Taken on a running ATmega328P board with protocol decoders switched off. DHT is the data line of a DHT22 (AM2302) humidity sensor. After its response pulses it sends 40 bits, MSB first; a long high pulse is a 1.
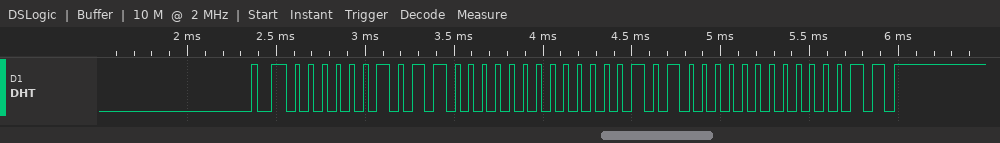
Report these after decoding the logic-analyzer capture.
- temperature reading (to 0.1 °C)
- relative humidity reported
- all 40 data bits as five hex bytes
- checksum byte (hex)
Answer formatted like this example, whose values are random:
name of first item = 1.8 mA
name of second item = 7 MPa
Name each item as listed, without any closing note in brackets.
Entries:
temperature reading = 32.0 °C
relative humidity reported = 70.4 %
all 40 data bits as five hex bytes = 02 C0 01 40 03
checksum byte = 0x03
